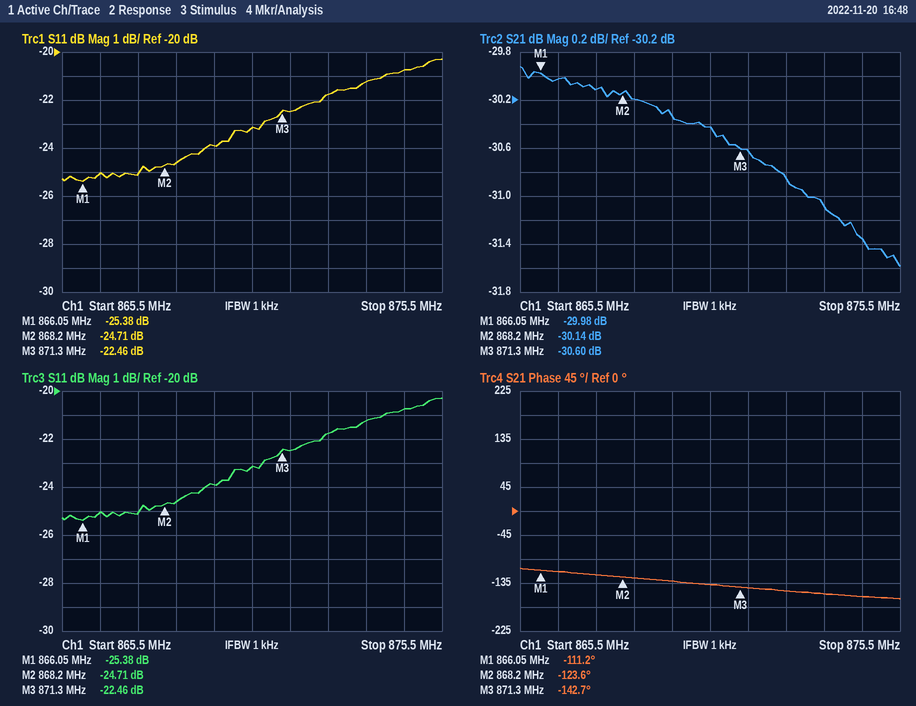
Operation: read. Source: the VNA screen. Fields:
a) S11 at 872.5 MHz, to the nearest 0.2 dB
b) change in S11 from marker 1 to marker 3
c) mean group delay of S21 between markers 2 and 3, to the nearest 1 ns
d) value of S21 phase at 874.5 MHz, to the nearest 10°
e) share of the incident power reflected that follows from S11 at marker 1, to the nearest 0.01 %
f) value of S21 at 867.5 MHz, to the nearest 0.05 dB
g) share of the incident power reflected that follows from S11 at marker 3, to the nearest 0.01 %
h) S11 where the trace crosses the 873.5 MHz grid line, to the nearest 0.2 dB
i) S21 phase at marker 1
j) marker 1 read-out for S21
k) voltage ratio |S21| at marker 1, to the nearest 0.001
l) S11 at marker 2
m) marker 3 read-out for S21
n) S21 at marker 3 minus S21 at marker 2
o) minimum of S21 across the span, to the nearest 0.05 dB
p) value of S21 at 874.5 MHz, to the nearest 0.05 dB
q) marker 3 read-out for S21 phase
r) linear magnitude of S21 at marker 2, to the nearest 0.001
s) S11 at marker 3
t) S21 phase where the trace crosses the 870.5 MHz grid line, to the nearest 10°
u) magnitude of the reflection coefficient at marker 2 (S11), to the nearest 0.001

-21.8 dB
2.92 dB
17 ns
-160°
0.29 %
-30.10 dB
0.57 %
-21.2 dB
-111.2°
-29.98 dB
0.032
-24.71 dB
-30.60 dB
-0.46 dB
-31.60 dB
-31.35 dB
-142.7°
0.031
-22.46 dB
-140°
0.058
